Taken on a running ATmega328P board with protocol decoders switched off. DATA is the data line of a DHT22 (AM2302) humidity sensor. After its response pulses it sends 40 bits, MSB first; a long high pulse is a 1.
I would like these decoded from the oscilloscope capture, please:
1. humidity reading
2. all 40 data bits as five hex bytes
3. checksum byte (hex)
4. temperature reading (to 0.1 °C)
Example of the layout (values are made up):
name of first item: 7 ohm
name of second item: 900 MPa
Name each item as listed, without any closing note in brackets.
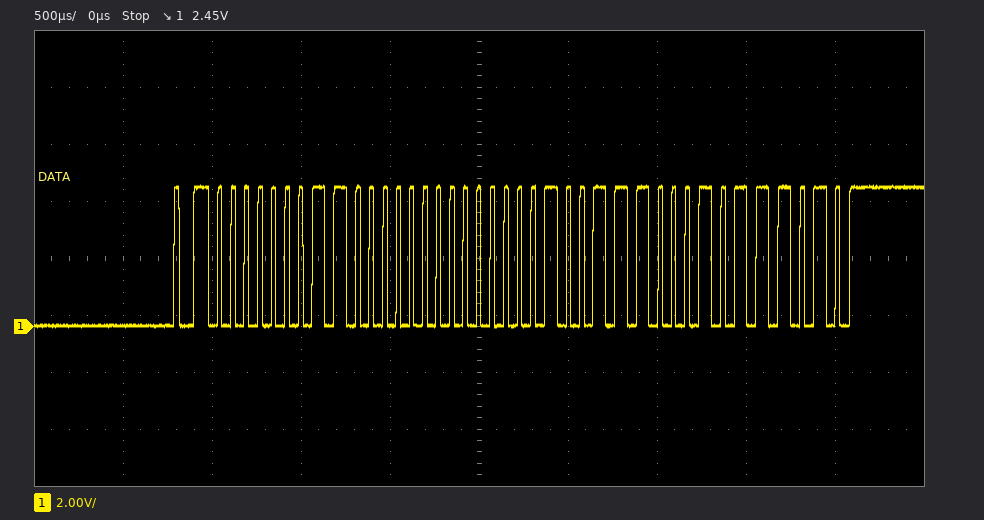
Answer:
humidity reading: 38.4 %
all 40 data bits as five hex bytes: 01 80 01 38 BA
checksum byte: 0xBA
temperature reading: 31.2 °C
